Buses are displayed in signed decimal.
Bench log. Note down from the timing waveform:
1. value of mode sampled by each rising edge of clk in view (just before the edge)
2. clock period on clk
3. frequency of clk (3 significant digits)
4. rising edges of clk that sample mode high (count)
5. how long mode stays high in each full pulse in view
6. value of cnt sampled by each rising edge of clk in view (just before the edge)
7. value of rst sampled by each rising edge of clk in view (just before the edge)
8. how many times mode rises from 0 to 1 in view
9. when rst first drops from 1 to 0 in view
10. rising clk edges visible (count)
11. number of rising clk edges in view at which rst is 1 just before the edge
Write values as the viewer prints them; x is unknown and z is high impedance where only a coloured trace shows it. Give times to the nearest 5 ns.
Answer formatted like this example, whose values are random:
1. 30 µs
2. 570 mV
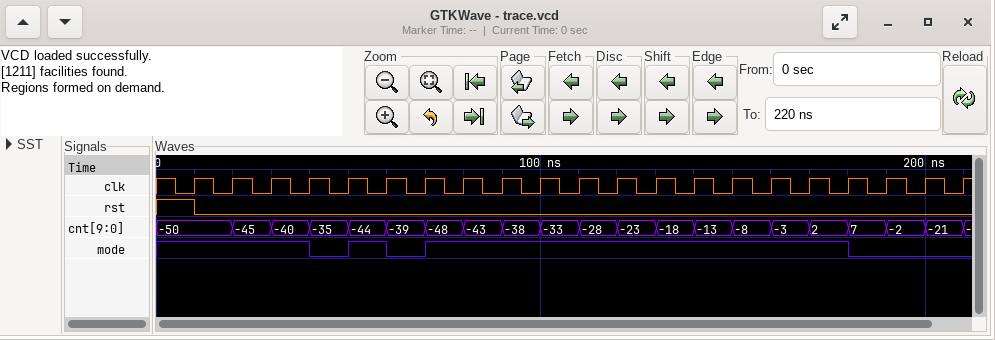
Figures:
1. 1 1 1 1 0 1 0 1 1 1 1 1 1 1 1 1 1 1 0 0 0
2. 10 ns
3. 100 MHz
4. 16
5. 10 ns, 110 ns
6. -50, -50, -45, -40, -35, -44, -39, -48, -43, -38, -33, -28, -23, -18, -13, -8, -3, 2, 7, -2, -21
7. 1 0 0 0 0 0 0 0 0 0 0 0 0 0 0 0 0 0 0 0 0
8. 2
9. 10 ns
10. 21
11. 1
